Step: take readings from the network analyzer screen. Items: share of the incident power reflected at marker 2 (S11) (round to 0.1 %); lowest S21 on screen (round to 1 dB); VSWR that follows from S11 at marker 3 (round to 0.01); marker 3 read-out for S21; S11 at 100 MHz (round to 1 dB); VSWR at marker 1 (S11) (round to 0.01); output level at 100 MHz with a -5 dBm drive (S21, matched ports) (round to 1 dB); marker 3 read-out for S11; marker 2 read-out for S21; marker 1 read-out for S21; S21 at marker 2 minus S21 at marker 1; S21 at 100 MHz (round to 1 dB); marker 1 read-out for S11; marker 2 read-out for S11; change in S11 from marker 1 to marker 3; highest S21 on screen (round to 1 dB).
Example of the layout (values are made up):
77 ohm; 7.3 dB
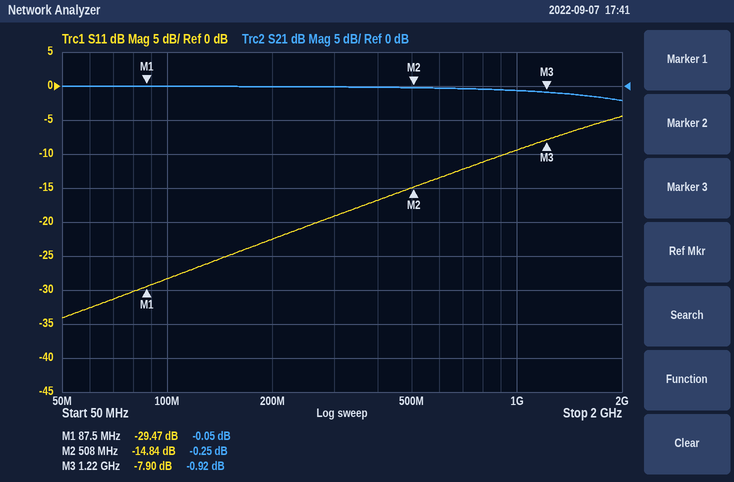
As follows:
3.3 %; -2 dB; 2.35; -0.92 dB; -28 dB; 1.07; -5 dBm; -7.90 dB; -0.25 dB; -0.05 dB; -0.20 dB; 0 dB; -29.47 dB; -14.84 dB; 21.57 dB; 0 dB
